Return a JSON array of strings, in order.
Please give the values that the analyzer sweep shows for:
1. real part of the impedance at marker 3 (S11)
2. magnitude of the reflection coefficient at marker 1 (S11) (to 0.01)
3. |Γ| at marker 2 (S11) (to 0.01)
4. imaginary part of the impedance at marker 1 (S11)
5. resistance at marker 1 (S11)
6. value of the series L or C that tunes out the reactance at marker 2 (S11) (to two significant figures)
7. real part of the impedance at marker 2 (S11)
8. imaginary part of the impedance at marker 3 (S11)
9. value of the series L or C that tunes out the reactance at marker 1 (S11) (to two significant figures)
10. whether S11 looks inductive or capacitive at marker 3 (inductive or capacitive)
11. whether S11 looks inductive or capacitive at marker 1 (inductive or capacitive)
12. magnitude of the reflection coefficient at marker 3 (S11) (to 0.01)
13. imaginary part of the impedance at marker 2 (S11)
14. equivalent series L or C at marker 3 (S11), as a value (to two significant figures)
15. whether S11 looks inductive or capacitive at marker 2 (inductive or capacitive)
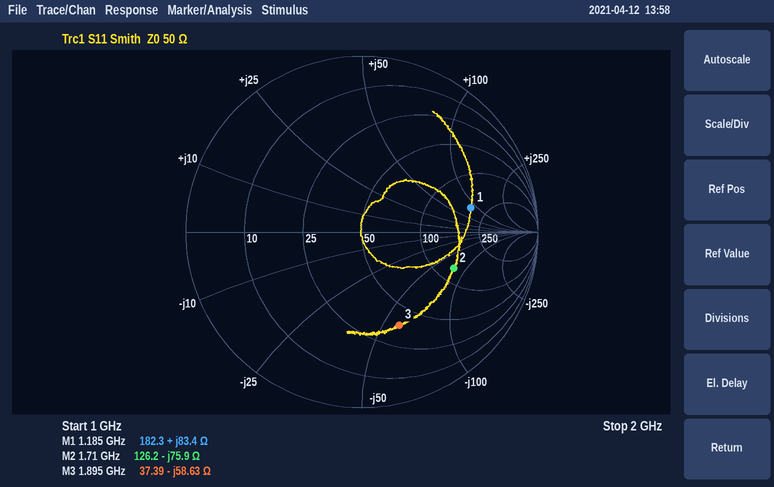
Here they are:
["37.39 Ω", "0.63", "0.56", "+83.4 Ω", "182.3 Ω", "7.1 nH", "126.2 Ω", "-58.63 Ω", "1.6 pF", "capacitive", "inductive", "0.57", "-75.9 Ω", "1.4 pF", "capacitive"]
